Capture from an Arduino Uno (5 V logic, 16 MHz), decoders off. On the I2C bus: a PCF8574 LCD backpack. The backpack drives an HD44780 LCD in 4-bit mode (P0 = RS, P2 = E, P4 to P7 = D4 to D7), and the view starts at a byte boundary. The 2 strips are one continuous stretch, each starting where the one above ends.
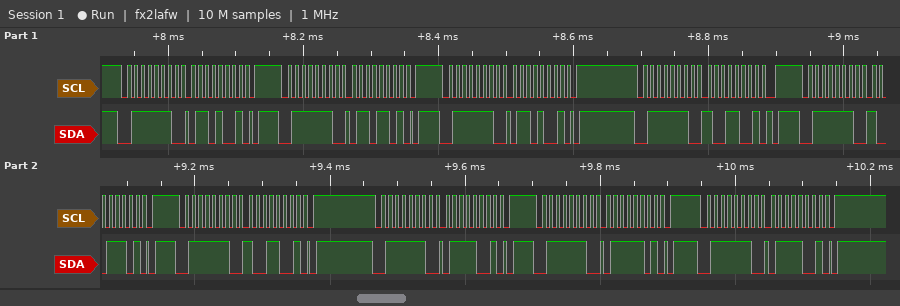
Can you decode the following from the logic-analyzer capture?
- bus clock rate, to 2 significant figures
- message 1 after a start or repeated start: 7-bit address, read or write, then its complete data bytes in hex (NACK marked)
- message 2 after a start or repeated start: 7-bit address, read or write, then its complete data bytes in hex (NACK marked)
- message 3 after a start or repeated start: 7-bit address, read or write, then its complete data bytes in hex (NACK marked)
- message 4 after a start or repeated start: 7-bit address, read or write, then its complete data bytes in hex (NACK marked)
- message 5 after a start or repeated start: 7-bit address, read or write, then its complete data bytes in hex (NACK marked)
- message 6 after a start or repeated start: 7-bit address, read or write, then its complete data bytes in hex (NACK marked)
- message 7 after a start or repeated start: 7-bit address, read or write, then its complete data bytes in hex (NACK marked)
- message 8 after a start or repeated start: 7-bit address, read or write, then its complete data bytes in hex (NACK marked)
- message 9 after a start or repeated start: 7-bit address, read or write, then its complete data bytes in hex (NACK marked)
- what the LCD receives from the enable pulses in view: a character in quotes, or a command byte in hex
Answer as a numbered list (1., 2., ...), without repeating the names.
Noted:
1. 100 kHz
2. 0x3F write: 69
3. 0x3F write: 6D
4. 0x3F write: 69
5. 0x3F write: 99
6. 0x3F write: 9D
7. 0x3F write: 99
8. 0x3F write: 79
9. 0x3F write: 7D
10. 0x3F write: 79
11. 'i'
